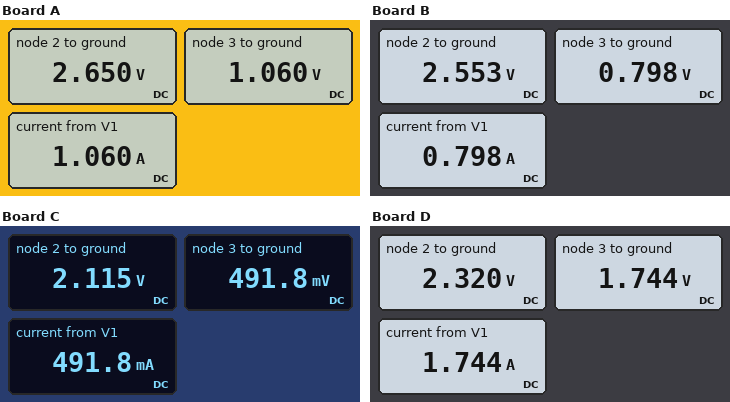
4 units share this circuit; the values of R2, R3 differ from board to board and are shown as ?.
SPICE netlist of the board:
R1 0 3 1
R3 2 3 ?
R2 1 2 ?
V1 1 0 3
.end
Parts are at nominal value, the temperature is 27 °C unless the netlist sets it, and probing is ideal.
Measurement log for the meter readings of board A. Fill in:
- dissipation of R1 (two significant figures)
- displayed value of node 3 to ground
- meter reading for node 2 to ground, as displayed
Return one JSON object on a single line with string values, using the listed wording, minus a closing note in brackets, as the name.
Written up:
{"dissipation of R1": "1.1 W", "displayed value of node 3 to ground": "1.060 V", "meter reading for node 2 to ground, as displayed": "2.650 V"}
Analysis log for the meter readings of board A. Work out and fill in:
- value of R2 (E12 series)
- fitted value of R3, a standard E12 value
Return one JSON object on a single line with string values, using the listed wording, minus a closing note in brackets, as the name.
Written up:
{"value of R2": "0.33 Ω", "fitted value of R3, a standard E12 value": "1.5 Ω"}
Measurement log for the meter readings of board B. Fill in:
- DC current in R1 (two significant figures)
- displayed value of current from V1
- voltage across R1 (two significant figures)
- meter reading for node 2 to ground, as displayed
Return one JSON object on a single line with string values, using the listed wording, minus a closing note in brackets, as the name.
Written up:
{"DC current in R1": "800 mA", "displayed value of current from V1": "0.798 A", "voltage across R1": "800 mV", "meter reading for node 2 to ground, as displayed": "2.553 V"}
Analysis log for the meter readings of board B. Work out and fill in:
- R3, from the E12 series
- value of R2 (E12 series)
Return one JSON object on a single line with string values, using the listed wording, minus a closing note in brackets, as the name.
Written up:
{"R3, from the E12 series": "2.2 Ω", "value of R2": "0.56 Ω"}
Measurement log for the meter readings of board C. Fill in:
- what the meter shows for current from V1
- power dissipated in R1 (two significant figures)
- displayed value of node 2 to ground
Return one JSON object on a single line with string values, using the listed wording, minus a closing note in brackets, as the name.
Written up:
{"what the meter shows for current from V1": "491.8 mA", "power dissipated in R1": "240 mW", "displayed value of node 2 to ground": "2.115 V"}
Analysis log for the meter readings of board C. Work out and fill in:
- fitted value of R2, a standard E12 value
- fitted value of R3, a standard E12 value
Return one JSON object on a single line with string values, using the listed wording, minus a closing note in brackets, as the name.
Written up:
{"fitted value of R2, a standard E12 value": "1.8 Ω", "fitted value of R3, a standard E12 value": "3.3 Ω"}
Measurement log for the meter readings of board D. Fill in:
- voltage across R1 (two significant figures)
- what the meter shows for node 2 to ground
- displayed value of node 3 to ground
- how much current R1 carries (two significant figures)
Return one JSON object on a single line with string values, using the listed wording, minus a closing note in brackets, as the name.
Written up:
{"voltage across R1": "1.7 V", "what the meter shows for node 2 to ground": "2.320 V", "displayed value of node 3 to ground": "1.744 V", "how much current R1 carries": "1.7 A"}
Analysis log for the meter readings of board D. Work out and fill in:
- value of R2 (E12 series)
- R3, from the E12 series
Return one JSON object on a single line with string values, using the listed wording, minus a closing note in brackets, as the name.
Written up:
{"value of R2": "0.39 Ω", "R3, from the E12 series": "0.33 Ω"}
